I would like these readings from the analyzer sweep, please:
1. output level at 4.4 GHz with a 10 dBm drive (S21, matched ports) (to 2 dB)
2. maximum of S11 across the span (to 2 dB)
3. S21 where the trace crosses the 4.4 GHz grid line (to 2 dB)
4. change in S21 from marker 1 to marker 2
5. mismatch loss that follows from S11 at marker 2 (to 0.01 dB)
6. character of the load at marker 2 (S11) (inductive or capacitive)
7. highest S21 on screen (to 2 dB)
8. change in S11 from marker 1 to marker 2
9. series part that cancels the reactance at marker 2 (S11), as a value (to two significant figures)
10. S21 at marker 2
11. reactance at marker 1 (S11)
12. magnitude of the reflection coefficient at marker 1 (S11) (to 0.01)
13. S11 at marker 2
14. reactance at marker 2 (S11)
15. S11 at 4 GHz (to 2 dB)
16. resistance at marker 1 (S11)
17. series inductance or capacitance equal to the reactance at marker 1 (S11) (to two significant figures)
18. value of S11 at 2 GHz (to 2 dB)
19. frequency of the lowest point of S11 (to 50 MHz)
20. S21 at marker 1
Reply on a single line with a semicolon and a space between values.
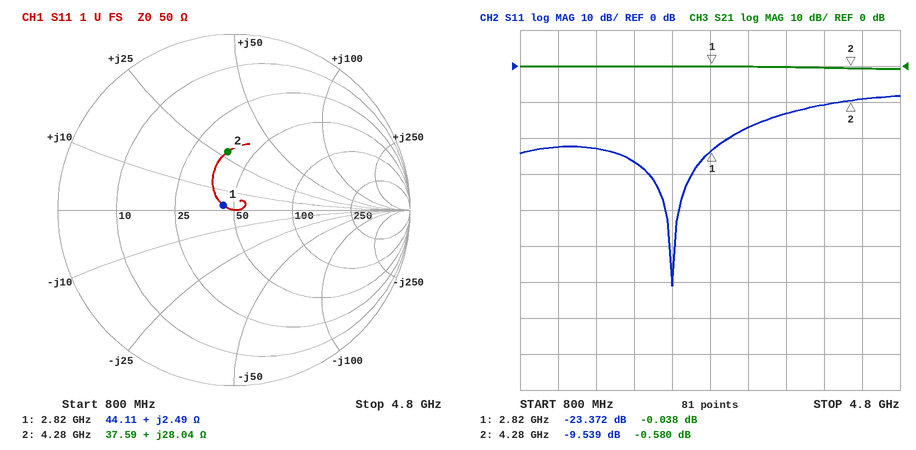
10 dBm; -8 dB; 0 dB; -0.542 dB; 0.51 dB; inductive; 0 dB; 13.833 dB; 1.3 pF; -0.580 dB; +2.49 Ω; 0.07; -9.539 dB; +28.04 Ω; -10 dB; 44.11 Ω; 140 pH; -26 dB; 2.40 GHz; -0.038 dB
